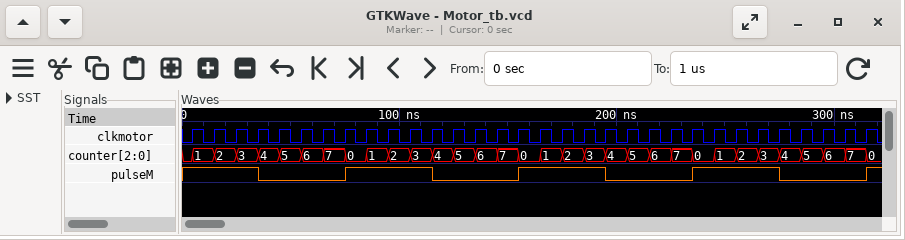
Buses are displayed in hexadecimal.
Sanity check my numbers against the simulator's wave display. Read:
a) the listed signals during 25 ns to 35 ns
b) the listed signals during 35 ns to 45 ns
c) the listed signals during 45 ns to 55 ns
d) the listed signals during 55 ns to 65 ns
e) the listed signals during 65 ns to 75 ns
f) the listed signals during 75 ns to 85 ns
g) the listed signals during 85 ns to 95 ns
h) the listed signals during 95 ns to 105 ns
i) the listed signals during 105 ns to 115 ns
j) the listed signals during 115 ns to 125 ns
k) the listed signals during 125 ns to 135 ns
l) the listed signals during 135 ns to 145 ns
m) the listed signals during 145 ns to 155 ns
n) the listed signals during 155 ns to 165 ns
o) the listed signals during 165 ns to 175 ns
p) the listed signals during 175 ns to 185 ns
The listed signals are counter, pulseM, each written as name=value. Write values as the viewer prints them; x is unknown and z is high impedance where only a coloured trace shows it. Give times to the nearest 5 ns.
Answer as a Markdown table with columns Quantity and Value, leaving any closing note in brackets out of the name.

| Quantity | Value |
|---|---|
| the listed signals during 25 ns to 35 ns | counter=3, pulseM=1 |
| the listed signals during 35 ns to 45 ns | counter=4, pulseM=0 |
| the listed signals during 45 ns to 55 ns | counter=5, pulseM=0 |
| the listed signals during 55 ns to 65 ns | counter=6, pulseM=0 |
| the listed signals during 65 ns to 75 ns | counter=7, pulseM=0 |
| the listed signals during 75 ns to 85 ns | counter=0, pulseM=1 |
| the listed signals during 85 ns to 95 ns | counter=1, pulseM=1 |
| the listed signals during 95 ns to 105 ns | counter=2, pulseM=1 |
| the listed signals during 105 ns to 115 ns | counter=3, pulseM=1 |
| the listed signals during 115 ns to 125 ns | counter=4, pulseM=0 |
| the listed signals during 125 ns to 135 ns | counter=5, pulseM=0 |
| the listed signals during 135 ns to 145 ns | counter=6, pulseM=0 |
| the listed signals during 145 ns to 155 ns | counter=7, pulseM=0 |
| the listed signals during 155 ns to 165 ns | counter=0, pulseM=1 |
| the listed signals during 165 ns to 175 ns | counter=1, pulseM=1 |
| the listed signals during 175 ns to 185 ns | counter=2, pulseM=1 |
